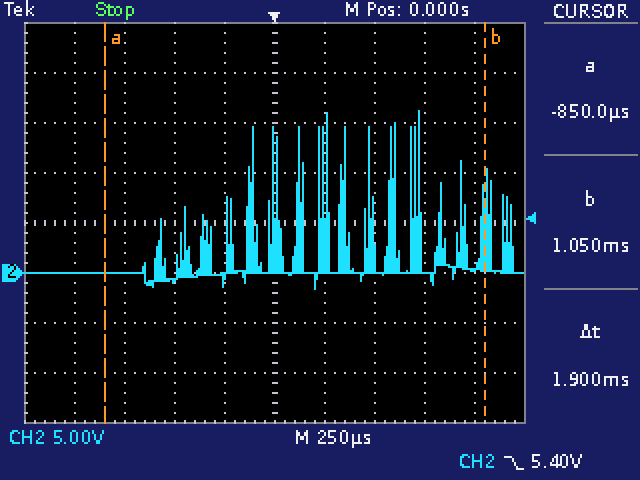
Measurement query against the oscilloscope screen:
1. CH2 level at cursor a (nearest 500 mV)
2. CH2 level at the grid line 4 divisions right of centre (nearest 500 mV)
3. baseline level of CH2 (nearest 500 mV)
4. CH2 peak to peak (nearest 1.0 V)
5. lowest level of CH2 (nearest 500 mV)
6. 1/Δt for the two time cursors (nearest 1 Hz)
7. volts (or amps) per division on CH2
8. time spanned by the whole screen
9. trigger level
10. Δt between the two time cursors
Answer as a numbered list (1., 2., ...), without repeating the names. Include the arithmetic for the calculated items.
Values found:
1. 0.0 V
2. 500 mV
3. 0.0 V
4. 18.0 V
5. -1.5 V
6. 1 / 1.9 ms ≈ 526 Hz
7. 5 V
8. 2.5 ms
9. 5.40 V
10. 1.9 ms
